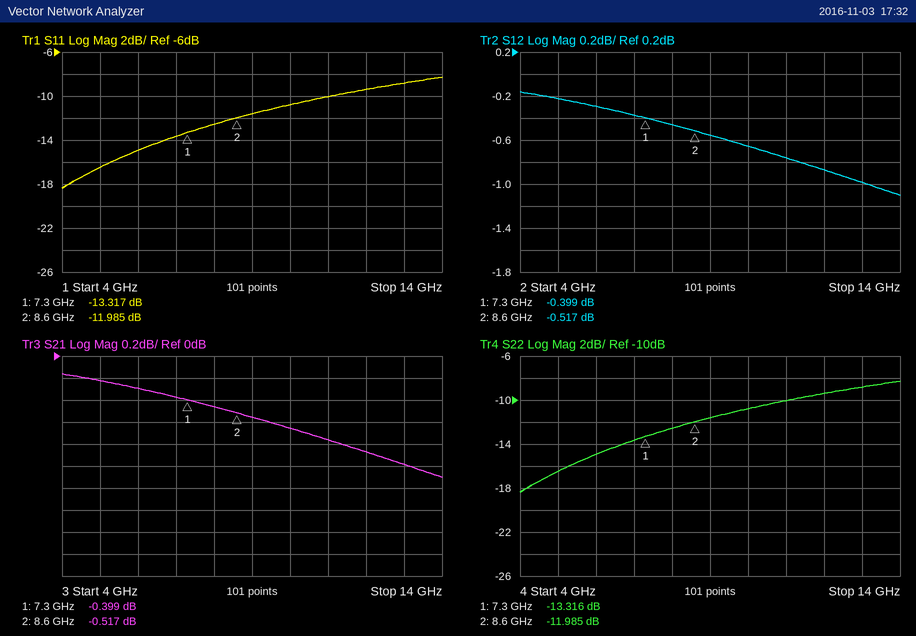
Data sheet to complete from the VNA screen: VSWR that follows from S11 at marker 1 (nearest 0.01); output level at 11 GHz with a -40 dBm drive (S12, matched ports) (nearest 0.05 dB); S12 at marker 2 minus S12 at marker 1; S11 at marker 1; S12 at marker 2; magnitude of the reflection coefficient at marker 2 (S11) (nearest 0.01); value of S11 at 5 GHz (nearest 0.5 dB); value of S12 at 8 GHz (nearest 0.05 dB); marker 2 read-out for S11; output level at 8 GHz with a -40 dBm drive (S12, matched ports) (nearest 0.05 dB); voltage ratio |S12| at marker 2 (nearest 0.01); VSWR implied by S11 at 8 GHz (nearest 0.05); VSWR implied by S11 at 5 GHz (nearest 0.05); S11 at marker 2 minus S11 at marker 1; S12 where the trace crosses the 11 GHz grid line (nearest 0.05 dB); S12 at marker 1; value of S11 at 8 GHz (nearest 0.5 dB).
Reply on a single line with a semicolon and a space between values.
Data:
1.55; -40.75 dBm; -0.118 dB; -13.317 dB; -0.517 dB; 0.25; -16.5 dB; -0.45 dB; -11.985 dB; -40.45 dBm; 0.94; 1.60; 1.35; 1.332 dB; -0.75 dB; -0.399 dB; -12.5 dB
